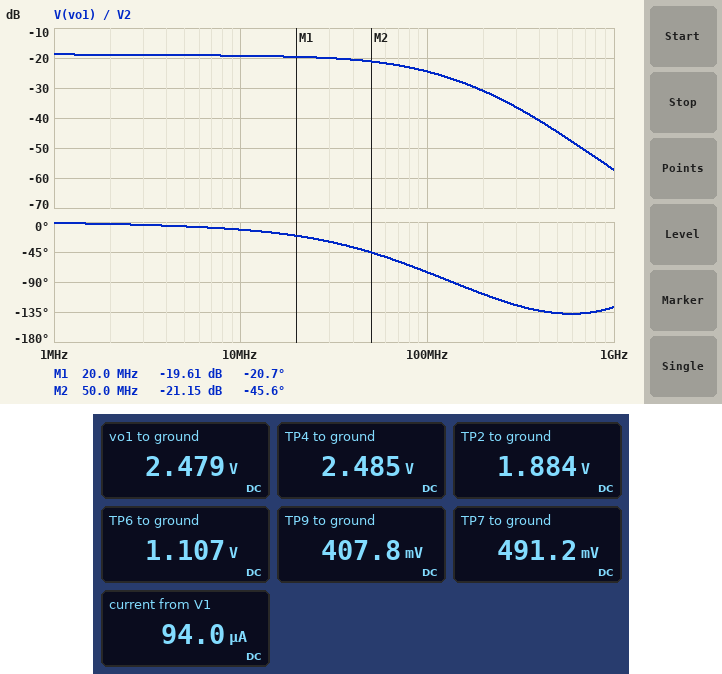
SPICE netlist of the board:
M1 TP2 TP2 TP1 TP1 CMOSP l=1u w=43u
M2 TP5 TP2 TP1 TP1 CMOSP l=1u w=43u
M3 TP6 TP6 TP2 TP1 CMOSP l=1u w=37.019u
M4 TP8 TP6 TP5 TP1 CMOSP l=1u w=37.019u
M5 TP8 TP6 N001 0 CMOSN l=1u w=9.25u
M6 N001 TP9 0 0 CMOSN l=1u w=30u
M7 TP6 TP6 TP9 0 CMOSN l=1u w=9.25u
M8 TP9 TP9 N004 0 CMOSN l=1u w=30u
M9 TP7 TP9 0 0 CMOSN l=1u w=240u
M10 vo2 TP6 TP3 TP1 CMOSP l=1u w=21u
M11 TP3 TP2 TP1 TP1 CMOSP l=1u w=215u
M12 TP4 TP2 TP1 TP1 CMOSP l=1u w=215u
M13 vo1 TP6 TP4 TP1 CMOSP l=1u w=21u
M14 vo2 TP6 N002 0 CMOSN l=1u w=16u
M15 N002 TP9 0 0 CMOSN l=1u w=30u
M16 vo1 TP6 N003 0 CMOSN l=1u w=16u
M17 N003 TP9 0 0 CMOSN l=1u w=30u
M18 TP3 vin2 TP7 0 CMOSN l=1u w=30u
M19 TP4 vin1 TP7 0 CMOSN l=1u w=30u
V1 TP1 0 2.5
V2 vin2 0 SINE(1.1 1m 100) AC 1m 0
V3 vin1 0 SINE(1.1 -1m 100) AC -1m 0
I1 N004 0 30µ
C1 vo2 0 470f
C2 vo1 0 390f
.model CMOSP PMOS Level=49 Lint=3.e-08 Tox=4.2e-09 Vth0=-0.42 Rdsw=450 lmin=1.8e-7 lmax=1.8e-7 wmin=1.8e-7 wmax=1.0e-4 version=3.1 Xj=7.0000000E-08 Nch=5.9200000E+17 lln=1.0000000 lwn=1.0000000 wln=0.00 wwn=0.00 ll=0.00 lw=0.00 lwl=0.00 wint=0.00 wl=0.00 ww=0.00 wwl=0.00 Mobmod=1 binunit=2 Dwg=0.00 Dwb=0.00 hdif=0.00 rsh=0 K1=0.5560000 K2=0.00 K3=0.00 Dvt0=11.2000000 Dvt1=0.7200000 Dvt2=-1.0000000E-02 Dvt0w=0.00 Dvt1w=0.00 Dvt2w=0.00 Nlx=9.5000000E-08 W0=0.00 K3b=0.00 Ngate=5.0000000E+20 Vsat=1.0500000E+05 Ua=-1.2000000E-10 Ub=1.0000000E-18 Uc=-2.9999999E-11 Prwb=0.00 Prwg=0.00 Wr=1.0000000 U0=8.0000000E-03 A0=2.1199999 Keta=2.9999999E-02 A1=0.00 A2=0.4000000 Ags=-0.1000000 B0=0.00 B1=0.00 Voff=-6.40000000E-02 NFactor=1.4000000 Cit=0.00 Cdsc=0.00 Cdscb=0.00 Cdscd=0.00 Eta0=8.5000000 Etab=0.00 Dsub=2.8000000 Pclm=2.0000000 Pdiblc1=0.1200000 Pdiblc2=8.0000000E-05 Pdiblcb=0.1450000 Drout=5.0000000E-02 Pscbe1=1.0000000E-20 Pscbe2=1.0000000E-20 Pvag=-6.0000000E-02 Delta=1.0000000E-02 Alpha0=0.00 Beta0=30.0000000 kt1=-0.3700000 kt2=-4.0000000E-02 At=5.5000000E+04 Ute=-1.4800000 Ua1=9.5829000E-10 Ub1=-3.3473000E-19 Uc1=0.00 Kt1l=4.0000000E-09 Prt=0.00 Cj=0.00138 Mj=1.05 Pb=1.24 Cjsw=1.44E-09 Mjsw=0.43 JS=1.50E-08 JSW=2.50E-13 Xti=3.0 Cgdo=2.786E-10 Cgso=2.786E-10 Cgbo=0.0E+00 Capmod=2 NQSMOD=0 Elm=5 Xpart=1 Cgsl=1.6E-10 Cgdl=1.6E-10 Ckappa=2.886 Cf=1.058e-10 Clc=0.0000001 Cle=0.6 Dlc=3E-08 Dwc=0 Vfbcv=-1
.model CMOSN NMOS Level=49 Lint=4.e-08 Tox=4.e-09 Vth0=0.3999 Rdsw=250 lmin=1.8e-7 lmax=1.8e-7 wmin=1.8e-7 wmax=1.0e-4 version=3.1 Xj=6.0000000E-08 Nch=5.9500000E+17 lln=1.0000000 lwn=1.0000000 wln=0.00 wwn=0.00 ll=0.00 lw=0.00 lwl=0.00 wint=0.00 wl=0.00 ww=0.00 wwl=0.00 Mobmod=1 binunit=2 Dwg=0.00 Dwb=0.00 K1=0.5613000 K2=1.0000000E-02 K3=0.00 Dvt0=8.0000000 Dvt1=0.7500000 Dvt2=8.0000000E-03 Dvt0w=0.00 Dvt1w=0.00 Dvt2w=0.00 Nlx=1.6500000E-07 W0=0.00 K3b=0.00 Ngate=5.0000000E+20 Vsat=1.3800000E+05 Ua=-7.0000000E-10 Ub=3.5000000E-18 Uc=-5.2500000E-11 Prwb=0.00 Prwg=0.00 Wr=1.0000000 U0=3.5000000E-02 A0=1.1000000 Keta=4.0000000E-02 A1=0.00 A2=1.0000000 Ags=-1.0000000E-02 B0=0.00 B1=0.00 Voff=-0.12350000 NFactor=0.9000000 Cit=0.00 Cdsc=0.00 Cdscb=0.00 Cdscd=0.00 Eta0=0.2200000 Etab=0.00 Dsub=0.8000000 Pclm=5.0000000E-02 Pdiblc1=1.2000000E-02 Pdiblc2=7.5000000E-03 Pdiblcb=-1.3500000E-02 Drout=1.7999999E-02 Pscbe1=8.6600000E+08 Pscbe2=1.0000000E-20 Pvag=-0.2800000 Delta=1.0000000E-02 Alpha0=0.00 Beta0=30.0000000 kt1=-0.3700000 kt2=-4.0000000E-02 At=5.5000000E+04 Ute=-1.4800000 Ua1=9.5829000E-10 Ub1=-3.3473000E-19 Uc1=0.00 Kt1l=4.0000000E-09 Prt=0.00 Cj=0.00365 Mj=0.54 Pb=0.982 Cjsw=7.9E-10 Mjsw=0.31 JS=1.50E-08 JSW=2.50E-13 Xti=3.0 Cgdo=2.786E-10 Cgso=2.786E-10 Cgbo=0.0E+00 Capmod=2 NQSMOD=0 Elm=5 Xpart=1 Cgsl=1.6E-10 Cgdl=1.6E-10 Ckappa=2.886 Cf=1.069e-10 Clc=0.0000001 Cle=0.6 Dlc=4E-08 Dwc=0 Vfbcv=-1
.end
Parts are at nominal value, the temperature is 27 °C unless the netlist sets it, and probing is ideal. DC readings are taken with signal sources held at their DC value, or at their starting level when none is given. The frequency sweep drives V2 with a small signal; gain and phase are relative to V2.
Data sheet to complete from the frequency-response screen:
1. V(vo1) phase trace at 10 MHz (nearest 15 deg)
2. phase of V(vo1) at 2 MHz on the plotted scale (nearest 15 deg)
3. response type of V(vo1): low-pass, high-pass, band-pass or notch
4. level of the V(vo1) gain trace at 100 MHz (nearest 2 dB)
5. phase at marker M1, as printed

-15 deg
0 deg
low-pass
-24 dB
-20.7 deg
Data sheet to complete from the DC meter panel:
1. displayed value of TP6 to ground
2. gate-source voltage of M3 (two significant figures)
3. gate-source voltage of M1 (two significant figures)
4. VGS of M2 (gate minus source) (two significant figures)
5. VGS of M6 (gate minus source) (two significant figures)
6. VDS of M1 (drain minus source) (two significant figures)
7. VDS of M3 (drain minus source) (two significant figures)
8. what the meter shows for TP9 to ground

1.107 V
-780 mV
-620 mV
-620 mV
410 mV
-620 mV
-780 mV
407.8 mV
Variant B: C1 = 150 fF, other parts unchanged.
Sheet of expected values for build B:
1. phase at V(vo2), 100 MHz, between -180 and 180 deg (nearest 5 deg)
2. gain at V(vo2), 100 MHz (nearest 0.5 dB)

130 deg
-21.0 dB
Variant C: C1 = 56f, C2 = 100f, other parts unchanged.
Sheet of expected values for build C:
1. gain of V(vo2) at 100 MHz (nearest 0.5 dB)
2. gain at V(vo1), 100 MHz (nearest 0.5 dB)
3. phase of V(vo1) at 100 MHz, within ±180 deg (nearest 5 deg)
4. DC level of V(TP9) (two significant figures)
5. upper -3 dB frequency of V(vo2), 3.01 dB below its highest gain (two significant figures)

-21.0 dB
-23.5 dB
-65 deg
410 mV
110 MHz
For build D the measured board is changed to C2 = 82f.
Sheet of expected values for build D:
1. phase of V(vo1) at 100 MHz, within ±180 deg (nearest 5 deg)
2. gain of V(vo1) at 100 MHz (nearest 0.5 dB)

-65 deg
-23.5 dB
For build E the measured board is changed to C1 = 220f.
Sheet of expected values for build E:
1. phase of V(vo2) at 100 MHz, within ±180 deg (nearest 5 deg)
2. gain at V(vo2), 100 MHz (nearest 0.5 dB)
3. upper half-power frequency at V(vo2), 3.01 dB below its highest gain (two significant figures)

125 deg
-21.5 dB
100 MHz
